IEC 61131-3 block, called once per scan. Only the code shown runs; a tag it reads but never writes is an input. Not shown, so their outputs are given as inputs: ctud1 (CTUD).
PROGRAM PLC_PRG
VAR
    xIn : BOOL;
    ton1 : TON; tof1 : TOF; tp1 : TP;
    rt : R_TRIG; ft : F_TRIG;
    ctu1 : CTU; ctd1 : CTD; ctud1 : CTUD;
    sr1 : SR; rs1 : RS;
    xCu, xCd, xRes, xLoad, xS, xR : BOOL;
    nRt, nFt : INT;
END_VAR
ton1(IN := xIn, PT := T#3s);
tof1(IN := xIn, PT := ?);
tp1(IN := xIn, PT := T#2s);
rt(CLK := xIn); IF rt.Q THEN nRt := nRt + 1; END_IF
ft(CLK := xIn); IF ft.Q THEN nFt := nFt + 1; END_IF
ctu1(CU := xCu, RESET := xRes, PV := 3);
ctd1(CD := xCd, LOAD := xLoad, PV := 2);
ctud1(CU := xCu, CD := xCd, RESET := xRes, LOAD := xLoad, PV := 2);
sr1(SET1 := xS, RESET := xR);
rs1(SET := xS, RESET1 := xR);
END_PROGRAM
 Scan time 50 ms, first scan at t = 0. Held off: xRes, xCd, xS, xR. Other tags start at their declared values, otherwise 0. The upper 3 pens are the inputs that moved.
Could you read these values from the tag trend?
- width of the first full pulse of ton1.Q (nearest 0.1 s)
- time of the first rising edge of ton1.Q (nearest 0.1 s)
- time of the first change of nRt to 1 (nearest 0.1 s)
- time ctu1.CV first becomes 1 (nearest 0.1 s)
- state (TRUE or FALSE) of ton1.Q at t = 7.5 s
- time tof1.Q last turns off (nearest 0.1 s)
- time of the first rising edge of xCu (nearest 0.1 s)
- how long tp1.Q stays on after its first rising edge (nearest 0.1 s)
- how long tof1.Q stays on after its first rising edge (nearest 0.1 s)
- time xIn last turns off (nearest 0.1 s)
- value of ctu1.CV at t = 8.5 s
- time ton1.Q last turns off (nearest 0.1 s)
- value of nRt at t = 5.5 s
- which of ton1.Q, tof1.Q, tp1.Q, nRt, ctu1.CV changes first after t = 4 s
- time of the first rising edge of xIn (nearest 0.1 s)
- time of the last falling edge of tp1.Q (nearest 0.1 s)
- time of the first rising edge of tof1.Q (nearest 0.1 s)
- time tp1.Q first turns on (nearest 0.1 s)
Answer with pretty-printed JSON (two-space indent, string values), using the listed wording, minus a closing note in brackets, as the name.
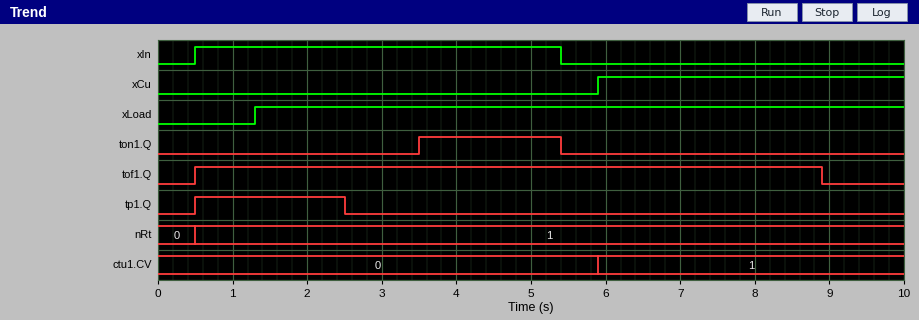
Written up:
{
  "width of the first full pulse of ton1.Q": "1.9 s",
  "time of the first rising edge of ton1.Q": "3.5 s",
  "time of the first change of nRt to 1": "0.5 s",
  "time ctu1.CV first becomes 1": "5.9 s",
  "state (TRUE or FALSE) of ton1.Q at t = 7.5 s": "FALSE",
  "time tof1.Q last turns off": "8.9 s",
  "time of the first rising edge of xCu": "5.9 s",
  "how long tp1.Q stays on after its first rising edge": "2.0 s",
  "how long tof1.Q stays on after its first rising edge": "8.4 s",
  "time xIn last turns off": "5.4 s",
  "value of ctu1.CV at t = 8.5 s": "1",
  "time ton1.Q last turns off": "5.4 s",
  "value of nRt at t = 5.5 s": "1",
  "which of ton1.Q, tof1.Q, tp1.Q, nRt, ctu1.CV changes first after t = 4 s": "ton1.Q",
  "time of the first rising edge of xIn": "0.5 s",
  "time of the last falling edge of tp1.Q": "2.5 s",
  "time of the first rising edge of tof1.Q": "0.5 s",
  "time tp1.Q first turns on": "0.5 s"
}
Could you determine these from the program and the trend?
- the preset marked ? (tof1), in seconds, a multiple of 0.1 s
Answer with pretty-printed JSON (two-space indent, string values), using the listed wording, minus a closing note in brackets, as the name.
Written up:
{
  "the preset marked ? (tof1), in seconds, a multiple of 0.1 s": "3.5 s"
}
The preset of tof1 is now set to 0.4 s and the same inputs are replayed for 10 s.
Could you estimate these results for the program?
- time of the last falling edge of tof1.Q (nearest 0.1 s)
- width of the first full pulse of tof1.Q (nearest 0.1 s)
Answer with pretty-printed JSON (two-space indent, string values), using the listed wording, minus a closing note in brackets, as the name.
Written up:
{
  "time of the last falling edge of tof1.Q": "5.8 s",
  "width of the first full pulse of tof1.Q": "5.3 s"
}
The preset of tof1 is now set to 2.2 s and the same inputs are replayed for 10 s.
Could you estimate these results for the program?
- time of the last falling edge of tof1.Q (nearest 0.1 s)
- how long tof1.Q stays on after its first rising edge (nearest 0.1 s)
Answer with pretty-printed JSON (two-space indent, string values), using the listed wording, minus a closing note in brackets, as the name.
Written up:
{
  "time of the last falling edge of tof1.Q": "7.6 s",
  "how long tof1.Q stays on after its first rising edge": "7.1 s"
}
